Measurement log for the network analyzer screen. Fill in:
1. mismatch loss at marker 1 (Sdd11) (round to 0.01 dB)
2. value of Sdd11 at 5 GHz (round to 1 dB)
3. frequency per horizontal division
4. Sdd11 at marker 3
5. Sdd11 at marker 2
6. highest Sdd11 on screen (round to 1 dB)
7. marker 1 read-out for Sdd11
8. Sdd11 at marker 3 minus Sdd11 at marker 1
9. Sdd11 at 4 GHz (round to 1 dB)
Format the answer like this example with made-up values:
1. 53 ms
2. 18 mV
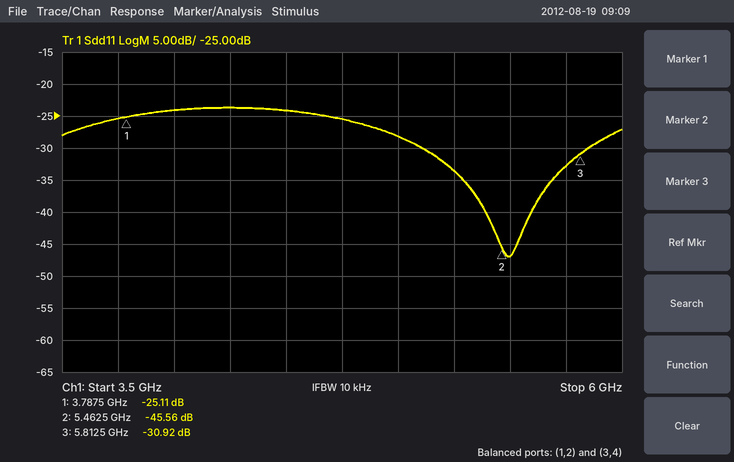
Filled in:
1. 0.01 dB
2. -28 dB
3. 250 MHz
4. -30.92 dB
5. -45.56 dB
6. -24 dB
7. -25.11 dB
8. -5.81 dB
9. -24 dB
